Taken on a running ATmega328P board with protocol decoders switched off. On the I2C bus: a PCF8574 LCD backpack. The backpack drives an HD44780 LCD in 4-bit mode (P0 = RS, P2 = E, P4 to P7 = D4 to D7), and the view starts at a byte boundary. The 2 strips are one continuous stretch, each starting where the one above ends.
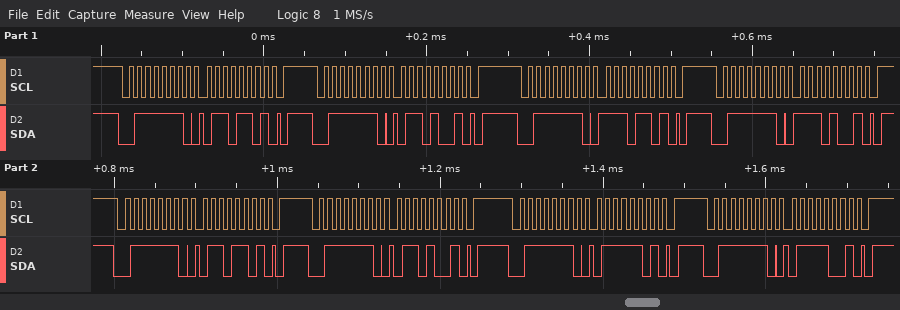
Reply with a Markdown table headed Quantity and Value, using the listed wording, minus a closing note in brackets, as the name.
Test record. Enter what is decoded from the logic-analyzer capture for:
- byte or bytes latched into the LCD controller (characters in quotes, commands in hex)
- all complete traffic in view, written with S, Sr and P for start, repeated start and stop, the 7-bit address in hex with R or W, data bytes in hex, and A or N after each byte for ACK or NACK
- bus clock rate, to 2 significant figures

| Quantity | Value |
|---|---|
| byte or bytes latched into the LCD controller | 'n' 'g' |
| all complete traffic in view, written with S, Sr and P for start, repeated start and stop, the 7-bit address in hex with R or W, data bytes in hex, and A or N after each byte for ACK or NACK | S 3FW A 6D A P S 3FW A 69 A P S 3FW A ED A P S 3FW A E9 A P S 3FW A 6D A P S 3FW A 69 A P S 3FW A 7D A P S 3FW A 79 A P |
| bus clock rate, to 2 significant figures | 100 kHz |
